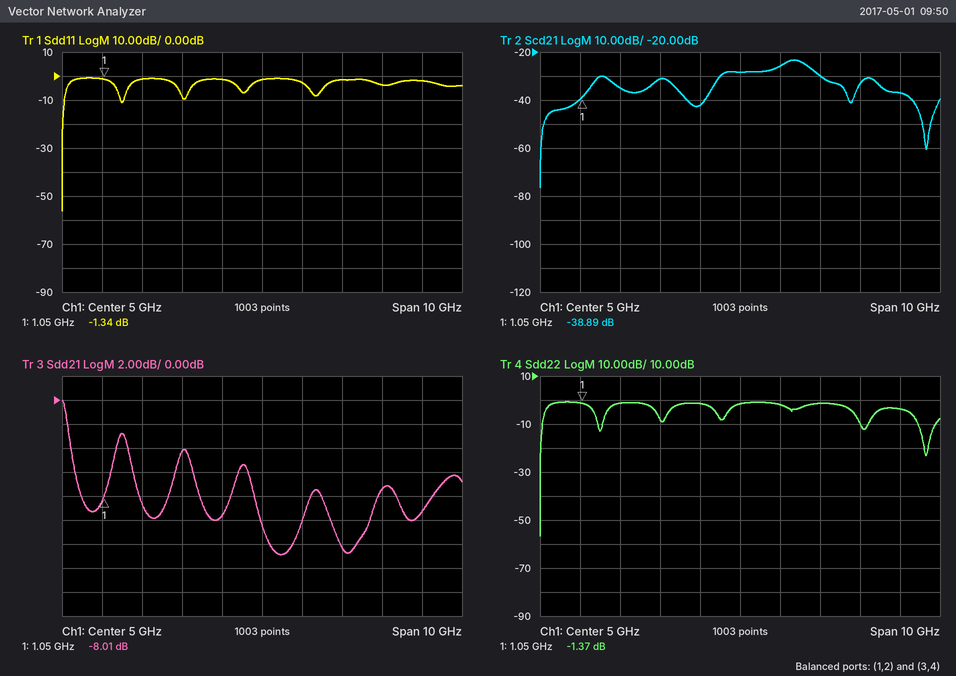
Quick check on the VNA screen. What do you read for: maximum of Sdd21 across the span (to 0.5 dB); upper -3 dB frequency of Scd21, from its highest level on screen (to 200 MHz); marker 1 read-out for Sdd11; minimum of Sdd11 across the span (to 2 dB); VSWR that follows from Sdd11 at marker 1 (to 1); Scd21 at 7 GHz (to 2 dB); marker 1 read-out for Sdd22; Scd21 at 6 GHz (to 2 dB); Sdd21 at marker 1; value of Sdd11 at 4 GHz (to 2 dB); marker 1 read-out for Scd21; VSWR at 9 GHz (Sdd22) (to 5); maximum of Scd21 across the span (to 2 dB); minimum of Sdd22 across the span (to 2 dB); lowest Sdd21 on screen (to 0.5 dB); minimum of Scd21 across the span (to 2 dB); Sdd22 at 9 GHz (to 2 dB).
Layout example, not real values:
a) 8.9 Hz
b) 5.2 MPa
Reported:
a) 0.0 dB
b) 6.8 GHz
c) -1.34 dB
d) -56 dB
e) 13
f) -30 dB
g) -1.37 dB
h) -26 dB
i) -8.01 dB
j) -2 dB
k) -38.89 dB
l) 5
m) -24 dB
n) -56 dB
o) -13.0 dB
p) -76 dB
q) -4 dB
